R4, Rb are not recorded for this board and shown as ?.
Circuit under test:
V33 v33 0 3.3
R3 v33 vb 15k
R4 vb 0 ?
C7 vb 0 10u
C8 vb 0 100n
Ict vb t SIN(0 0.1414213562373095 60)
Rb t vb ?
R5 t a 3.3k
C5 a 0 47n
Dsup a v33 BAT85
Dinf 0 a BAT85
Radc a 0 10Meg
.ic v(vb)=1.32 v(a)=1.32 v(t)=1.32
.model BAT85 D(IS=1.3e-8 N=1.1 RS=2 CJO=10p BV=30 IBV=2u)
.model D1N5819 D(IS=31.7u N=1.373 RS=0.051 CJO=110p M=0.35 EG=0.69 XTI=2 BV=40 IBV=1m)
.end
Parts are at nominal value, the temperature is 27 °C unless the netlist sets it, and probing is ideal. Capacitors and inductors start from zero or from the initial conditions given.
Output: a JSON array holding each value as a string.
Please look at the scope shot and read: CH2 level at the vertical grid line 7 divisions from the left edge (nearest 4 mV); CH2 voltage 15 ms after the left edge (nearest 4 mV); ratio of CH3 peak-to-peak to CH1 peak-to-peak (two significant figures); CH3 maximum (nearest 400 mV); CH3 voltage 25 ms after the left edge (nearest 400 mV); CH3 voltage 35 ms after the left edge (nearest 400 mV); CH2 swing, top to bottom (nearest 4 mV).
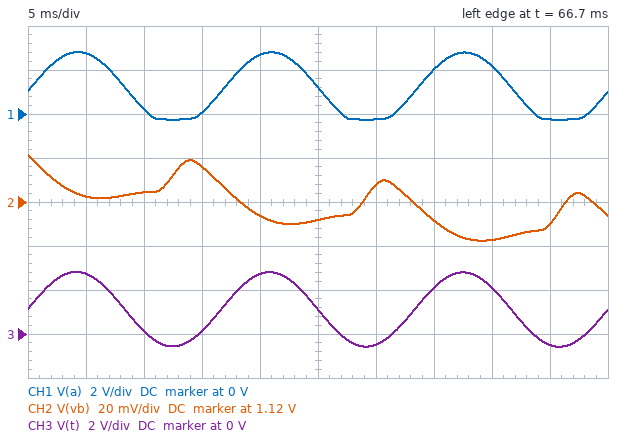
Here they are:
["1.112 V", "1.136 V", "1.1", "2.8 V", "1.2 V", "2.0 V", "40 mV"]
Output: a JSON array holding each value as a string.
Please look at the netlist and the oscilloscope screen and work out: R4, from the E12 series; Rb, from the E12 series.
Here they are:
["6.8 kΩ", "12 Ω"]
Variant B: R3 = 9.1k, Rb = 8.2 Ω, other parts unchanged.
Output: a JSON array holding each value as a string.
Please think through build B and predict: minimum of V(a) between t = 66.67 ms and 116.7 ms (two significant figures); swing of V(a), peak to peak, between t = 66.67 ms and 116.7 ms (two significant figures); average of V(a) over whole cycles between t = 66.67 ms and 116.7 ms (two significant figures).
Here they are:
["250 mV", "2.3 V", "1.4 V"]
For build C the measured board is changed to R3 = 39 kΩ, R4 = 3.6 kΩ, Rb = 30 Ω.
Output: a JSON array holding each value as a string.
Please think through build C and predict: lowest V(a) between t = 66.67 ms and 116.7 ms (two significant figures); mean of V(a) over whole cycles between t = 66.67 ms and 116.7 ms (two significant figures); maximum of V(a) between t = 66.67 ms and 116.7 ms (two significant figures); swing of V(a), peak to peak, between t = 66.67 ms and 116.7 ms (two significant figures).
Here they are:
["-320 mV", "1.4 V", "3.6 V", "3.9 V"]
